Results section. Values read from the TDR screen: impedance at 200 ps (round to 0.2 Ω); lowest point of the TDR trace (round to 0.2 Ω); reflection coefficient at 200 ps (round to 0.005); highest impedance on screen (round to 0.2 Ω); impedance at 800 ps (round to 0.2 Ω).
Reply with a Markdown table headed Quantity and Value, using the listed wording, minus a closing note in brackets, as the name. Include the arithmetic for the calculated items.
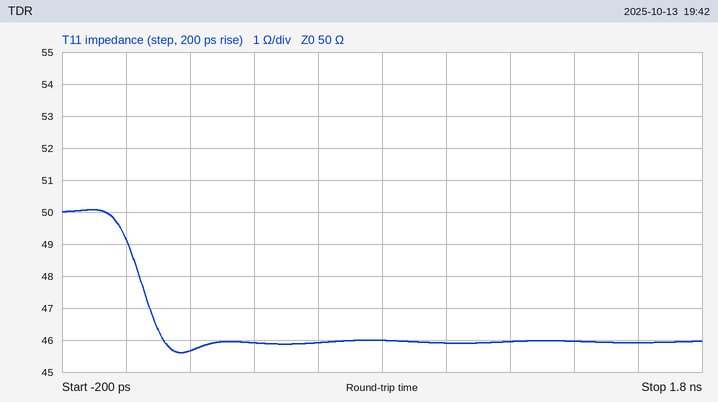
| Quantity | Value |
|---|---|
| impedance at 200 ps | 45.6 Ω |
| lowest point of the TDR trace | 45.6 Ω |
| reflection coefficient at 200 ps | (45.6 − 50)/(45.6 + 50) ≈ -0.0460, so -0.045 to the nearest 0.005 |
| highest impedance on screen | 50.0 Ω |
| impedance at 800 ps | 46.0 Ω |
